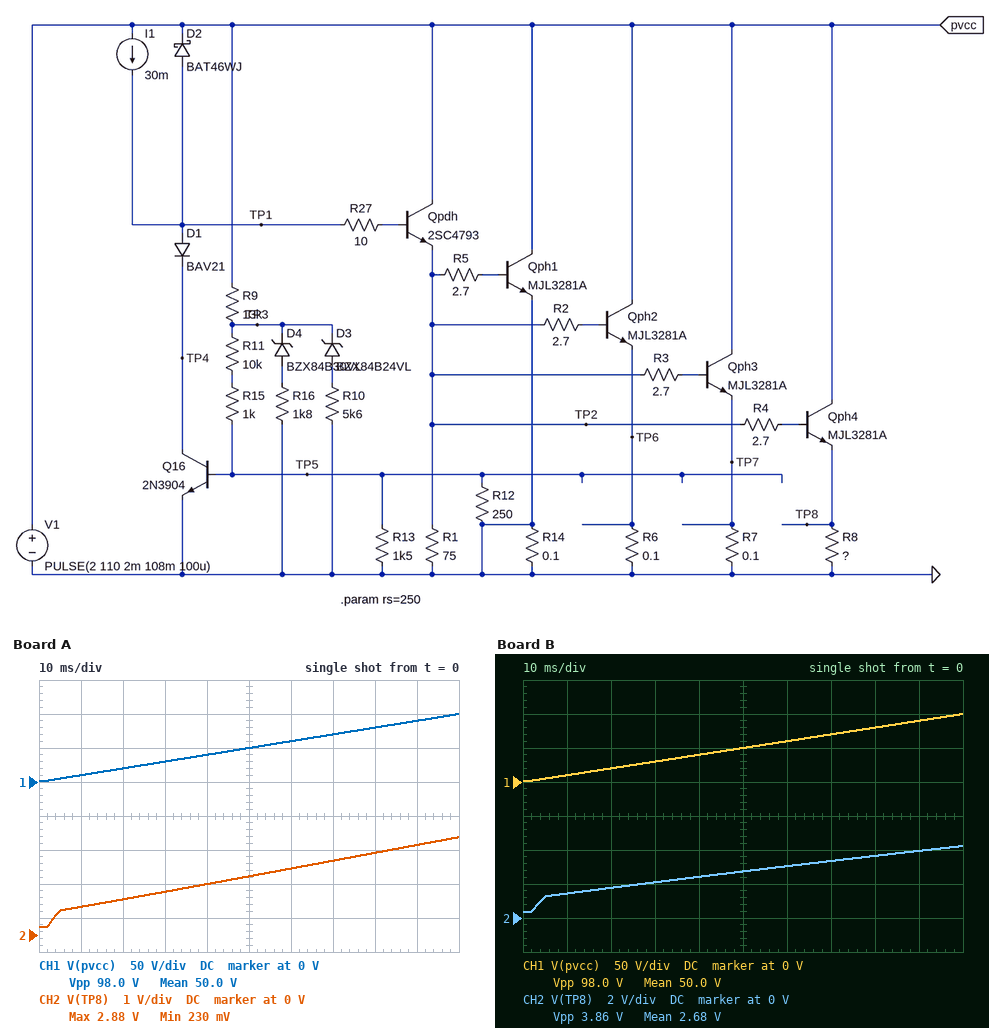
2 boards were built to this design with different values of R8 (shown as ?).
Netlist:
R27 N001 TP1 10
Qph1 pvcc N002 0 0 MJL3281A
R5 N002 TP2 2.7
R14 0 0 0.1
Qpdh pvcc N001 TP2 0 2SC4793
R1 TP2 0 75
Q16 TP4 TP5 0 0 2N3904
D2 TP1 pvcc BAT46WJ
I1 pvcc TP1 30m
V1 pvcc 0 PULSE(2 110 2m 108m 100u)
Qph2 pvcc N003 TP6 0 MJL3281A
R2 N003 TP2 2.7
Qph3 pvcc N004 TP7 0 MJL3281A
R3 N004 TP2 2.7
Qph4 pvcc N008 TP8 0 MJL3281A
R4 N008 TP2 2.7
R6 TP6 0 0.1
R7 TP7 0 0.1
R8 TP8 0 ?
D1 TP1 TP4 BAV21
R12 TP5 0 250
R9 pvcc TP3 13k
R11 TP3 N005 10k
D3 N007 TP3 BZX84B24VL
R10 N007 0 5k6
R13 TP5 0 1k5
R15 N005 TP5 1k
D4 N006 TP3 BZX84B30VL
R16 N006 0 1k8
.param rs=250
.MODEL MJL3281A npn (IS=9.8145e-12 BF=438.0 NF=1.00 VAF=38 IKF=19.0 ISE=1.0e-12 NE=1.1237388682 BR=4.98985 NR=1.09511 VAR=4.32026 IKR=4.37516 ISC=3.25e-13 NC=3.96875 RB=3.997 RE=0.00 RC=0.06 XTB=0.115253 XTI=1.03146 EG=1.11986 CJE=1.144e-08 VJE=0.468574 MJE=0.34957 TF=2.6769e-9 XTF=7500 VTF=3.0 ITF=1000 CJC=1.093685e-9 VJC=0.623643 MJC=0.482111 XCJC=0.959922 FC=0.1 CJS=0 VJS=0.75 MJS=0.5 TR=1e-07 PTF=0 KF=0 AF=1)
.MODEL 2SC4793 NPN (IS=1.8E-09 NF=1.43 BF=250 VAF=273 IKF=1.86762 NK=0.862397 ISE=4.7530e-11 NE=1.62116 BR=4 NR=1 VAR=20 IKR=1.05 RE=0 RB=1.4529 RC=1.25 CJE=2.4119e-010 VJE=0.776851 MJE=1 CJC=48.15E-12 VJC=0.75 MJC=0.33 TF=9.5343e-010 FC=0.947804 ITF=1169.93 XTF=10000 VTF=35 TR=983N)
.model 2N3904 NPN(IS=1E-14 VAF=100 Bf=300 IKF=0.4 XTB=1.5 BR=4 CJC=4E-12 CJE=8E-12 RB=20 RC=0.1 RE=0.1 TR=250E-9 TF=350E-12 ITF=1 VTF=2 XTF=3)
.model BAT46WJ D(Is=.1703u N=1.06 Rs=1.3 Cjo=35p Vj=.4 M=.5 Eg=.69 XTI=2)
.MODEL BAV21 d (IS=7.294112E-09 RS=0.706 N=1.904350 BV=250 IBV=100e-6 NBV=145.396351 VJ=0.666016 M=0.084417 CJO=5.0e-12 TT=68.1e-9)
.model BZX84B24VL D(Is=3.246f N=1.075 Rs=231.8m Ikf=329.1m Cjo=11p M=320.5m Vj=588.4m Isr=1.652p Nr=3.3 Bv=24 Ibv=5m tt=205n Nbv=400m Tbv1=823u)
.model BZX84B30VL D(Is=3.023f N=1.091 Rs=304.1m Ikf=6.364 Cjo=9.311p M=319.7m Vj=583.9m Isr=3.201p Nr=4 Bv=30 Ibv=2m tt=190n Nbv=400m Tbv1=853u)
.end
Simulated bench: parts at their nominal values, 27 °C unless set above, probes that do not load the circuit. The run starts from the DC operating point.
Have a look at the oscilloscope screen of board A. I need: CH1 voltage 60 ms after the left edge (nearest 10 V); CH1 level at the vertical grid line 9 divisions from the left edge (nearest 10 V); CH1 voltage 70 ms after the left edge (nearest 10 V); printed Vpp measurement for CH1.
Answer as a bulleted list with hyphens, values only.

- 60 V
- 90 V
- 70 V
- 98.0 V
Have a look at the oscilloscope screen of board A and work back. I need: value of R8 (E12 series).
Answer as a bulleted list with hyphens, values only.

- 0.039 Ω
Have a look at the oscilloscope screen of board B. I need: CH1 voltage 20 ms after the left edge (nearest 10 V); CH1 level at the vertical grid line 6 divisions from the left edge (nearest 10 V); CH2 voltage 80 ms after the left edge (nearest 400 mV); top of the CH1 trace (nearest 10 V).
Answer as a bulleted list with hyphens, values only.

- 20 V
- 60 V
- 3.6 V
- 100 V
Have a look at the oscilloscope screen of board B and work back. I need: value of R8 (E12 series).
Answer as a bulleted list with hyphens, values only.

- 0.082 Ω
